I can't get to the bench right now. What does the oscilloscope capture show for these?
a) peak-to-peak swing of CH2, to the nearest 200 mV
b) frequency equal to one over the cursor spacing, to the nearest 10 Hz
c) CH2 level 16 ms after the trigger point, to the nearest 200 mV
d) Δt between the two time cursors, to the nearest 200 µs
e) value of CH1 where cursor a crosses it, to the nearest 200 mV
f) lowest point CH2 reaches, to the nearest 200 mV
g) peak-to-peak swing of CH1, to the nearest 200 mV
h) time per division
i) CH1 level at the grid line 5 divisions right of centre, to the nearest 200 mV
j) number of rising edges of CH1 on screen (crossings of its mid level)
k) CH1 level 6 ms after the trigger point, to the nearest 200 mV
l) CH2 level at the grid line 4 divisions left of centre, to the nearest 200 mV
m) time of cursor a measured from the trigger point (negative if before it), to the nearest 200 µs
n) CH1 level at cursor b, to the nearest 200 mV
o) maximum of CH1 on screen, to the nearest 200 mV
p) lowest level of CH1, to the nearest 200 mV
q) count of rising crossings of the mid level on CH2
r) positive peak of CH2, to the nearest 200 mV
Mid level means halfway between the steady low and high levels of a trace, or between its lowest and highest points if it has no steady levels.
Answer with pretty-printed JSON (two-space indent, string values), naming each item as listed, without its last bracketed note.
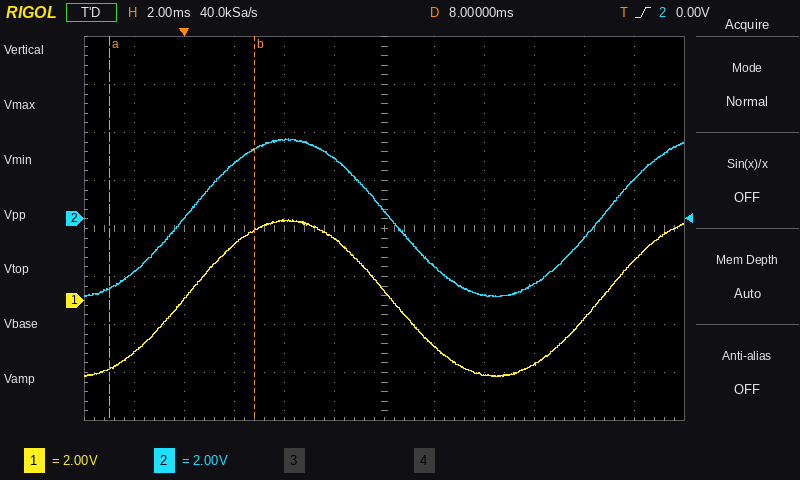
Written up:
{
  "peak-to-peak swing of CH2, to the nearest 200 mV": "6.6 V",
  "frequency equal to one over the cursor spacing, to the nearest 10 Hz": "170 Hz",
  "CH2 level 16 ms after the trigger point, to the nearest 200 mV": "-800 mV",
  "Δt between the two time cursors, to the nearest 200 µs": "5.8 ms",
  "value of CH1 where cursor a crosses it, to the nearest 200 mV": "-2.8 V",
  "lowest point CH2 reaches, to the nearest 200 mV": "-3.2 V",
  "peak-to-peak swing of CH1, to the nearest 200 mV": "6.6 V",
  "time per division": "2 ms",
  "CH1 level at the grid line 5 divisions right of centre, to the nearest 200 mV": "1.6 V",
  "number of rising edges of CH1 on screen": "2",
  "CH1 level 6 ms after the trigger point, to the nearest 200 mV": "2.6 V",
  "CH2 level at the grid line 4 divisions left of centre, to the nearest 200 mV": "0.0 V",
  "time of cursor a measured from the trigger point (negative if before it), to the nearest 200 µs": "-3.0 ms",
  "CH1 level at cursor b, to the nearest 200 mV": "3.0 V",
  "maximum of CH1 on screen, to the nearest 200 mV": "3.4 V",
  "lowest level of CH1, to the nearest 200 mV": "-3.2 V",
  "count of rising crossings of the mid level on CH2": "2",
  "positive peak of CH2, to the nearest 200 mV": "3.4 V"
}
